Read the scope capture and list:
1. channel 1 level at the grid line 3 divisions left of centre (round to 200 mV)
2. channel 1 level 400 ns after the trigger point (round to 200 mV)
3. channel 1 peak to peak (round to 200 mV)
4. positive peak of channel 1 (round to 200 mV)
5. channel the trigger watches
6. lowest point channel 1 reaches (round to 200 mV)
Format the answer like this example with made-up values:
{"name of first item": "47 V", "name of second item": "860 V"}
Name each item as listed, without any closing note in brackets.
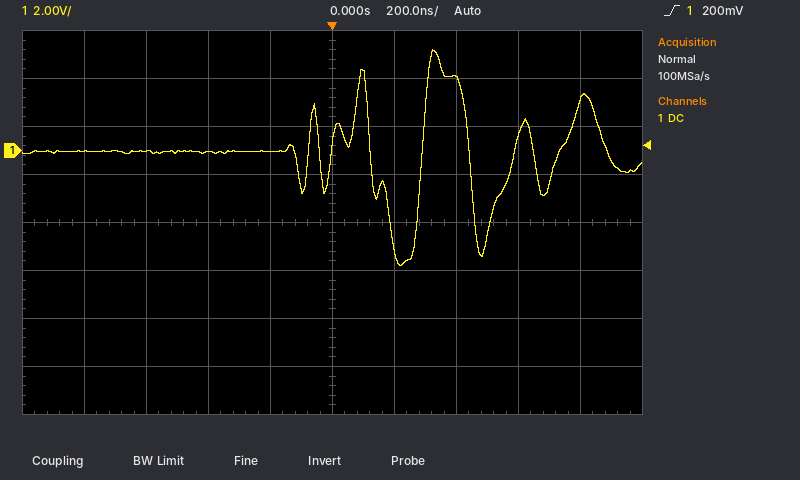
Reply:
{"channel 1 level at the grid line 3 divisions left of centre": "0.0 V", "channel 1 level 400 ns after the trigger point": "3.0 V", "channel 1 peak to peak": "9.0 V", "positive peak of channel 1": "4.2 V", "channel the trigger watches": "channel 1", "lowest point channel 1 reaches": "-4.8 V"}
